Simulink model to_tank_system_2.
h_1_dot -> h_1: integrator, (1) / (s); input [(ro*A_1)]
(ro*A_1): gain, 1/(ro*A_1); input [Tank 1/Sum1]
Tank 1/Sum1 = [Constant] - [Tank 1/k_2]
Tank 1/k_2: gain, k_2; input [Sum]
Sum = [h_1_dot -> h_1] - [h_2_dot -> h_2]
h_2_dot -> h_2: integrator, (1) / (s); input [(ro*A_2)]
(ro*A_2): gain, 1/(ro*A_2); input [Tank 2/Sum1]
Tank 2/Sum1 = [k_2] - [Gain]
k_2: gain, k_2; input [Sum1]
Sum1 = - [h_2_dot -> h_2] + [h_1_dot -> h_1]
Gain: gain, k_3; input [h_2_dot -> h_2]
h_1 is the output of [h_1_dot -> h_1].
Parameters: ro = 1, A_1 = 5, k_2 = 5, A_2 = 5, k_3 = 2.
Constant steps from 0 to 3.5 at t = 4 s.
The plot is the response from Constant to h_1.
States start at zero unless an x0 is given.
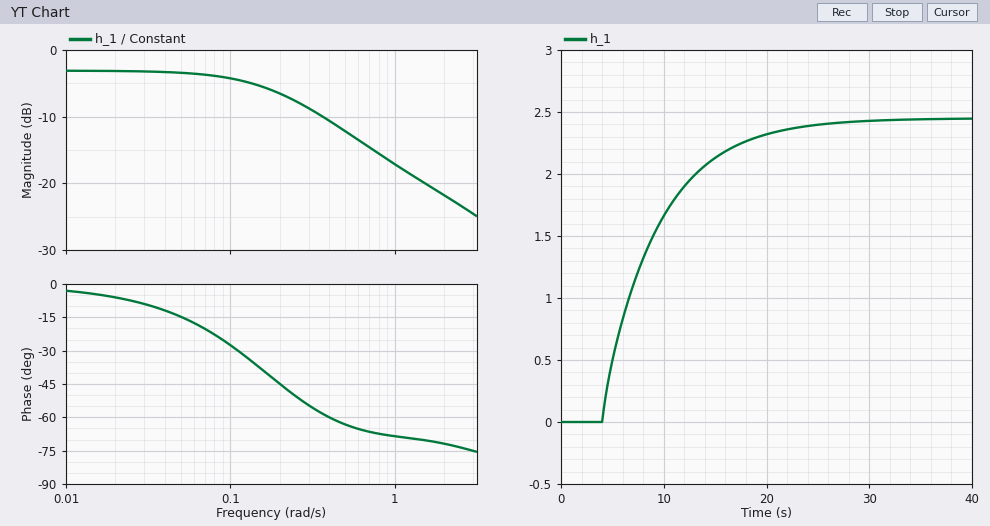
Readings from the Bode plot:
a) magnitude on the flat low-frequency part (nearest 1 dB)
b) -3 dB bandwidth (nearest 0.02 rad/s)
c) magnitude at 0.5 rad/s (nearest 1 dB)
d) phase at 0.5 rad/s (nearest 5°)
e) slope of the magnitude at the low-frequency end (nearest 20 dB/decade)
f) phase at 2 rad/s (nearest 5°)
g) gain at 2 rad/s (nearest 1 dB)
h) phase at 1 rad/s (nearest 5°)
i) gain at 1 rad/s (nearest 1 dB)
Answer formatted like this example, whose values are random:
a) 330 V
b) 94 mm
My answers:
a) -3 dB
b) 0.18 rad/s
c) -12 dB
d) -65°
e) 0 dB/decade
f) -70°
g) -22 dB
h) -70°
i) -17 dB
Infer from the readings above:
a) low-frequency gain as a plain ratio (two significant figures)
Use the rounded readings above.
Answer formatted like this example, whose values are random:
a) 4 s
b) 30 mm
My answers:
a) 0.71
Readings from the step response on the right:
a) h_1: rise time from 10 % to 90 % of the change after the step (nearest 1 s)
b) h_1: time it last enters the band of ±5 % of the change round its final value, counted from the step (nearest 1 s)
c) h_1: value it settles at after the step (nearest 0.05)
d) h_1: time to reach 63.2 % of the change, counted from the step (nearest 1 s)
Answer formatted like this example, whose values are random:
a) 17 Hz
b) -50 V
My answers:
a) 12 s
b) 16 s
c) 2.45
d) 5 s
